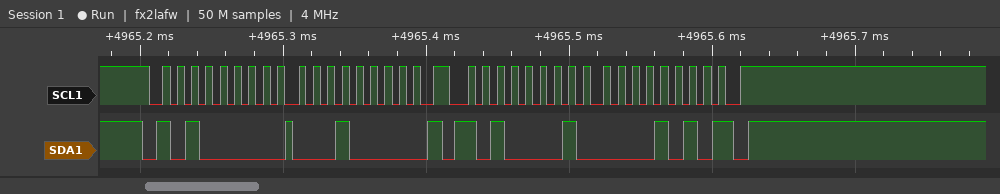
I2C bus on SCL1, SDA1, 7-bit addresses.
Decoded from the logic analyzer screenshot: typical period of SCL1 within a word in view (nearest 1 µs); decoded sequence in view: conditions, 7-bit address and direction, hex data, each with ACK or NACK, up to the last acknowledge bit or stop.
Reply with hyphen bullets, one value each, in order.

- 10 µs
- start, address 50 write ACK, 10 ACK, repeated start, address 50 read ACK, 0A NACK, stop
